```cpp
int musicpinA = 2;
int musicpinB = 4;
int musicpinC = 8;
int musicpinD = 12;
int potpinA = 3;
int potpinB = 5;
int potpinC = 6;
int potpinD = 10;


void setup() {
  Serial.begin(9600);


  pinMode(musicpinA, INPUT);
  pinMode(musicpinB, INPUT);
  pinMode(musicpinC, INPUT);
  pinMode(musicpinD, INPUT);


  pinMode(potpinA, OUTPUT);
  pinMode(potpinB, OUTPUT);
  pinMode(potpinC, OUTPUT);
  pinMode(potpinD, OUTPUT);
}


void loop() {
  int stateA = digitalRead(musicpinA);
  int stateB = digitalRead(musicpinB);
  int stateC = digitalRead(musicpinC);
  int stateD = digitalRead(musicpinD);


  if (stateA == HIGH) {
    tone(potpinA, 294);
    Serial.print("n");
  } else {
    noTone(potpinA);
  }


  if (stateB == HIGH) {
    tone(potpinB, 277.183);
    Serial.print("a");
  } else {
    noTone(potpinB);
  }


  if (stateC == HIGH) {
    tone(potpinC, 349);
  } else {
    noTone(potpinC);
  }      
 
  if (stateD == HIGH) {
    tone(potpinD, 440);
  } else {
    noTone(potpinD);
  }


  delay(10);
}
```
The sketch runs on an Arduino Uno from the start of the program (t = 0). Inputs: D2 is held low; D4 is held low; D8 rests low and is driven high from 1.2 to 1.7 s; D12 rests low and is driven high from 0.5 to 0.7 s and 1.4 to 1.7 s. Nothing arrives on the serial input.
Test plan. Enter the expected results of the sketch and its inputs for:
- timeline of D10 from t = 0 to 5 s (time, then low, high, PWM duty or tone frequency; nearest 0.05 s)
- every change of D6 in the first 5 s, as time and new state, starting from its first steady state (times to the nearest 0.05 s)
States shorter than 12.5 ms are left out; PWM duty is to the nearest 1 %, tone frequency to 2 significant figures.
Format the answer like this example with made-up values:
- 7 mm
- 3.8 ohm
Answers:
- 0 s low; 0.5 s tone 440 Hz; 0.7 s low
- 0 s low; 1.2 s tone 350 Hz; 1.7 s low
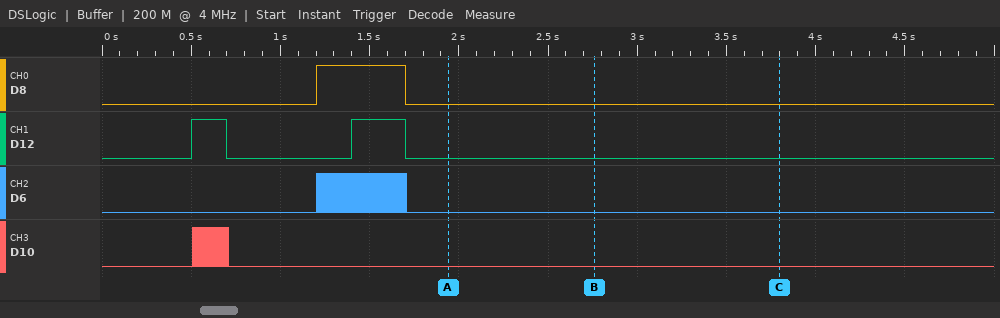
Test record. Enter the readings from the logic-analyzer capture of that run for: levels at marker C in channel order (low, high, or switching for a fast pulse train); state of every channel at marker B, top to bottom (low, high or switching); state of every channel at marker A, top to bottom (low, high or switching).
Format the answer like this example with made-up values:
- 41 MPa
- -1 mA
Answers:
- D8 low, D12 low, D6 low, D10 low
- D8 low, D12 low, D6 low, D10 low
- D8 low, D12 low, D6 low, D10 low
